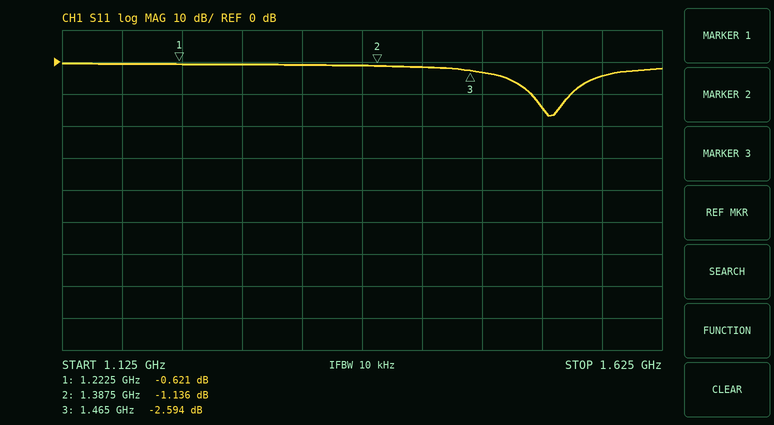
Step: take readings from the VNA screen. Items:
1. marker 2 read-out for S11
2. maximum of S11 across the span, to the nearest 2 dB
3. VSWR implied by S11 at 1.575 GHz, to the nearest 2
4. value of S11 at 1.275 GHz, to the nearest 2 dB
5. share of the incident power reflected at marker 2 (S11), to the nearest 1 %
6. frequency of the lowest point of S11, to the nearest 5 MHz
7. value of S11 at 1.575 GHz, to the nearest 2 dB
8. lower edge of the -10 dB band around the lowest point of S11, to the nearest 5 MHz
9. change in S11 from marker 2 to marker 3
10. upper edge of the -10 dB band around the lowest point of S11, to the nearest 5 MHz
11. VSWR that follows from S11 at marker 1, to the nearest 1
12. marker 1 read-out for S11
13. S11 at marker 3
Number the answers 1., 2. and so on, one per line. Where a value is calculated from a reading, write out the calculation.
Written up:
1. -1.136 dB
2. 0 dB
3. |Γ| = 10^(-4/20) = 0.6310; VSWR = (1 + 0.6310)/(1 − 0.6310) ≈ 4
4. 0 dB
5. 10^(-1.136/10) ≈ 77 %
6. 1.530 GHz
7. -4 dB
8. 1.515 GHz
9. -2.594 − (-1.136) = -1.458 dB
10. 1.550 GHz
11. (1 + 0.9310)/(1 − 0.9310) ≈ 28
12. -0.621 dB
13. -2.594 dB
